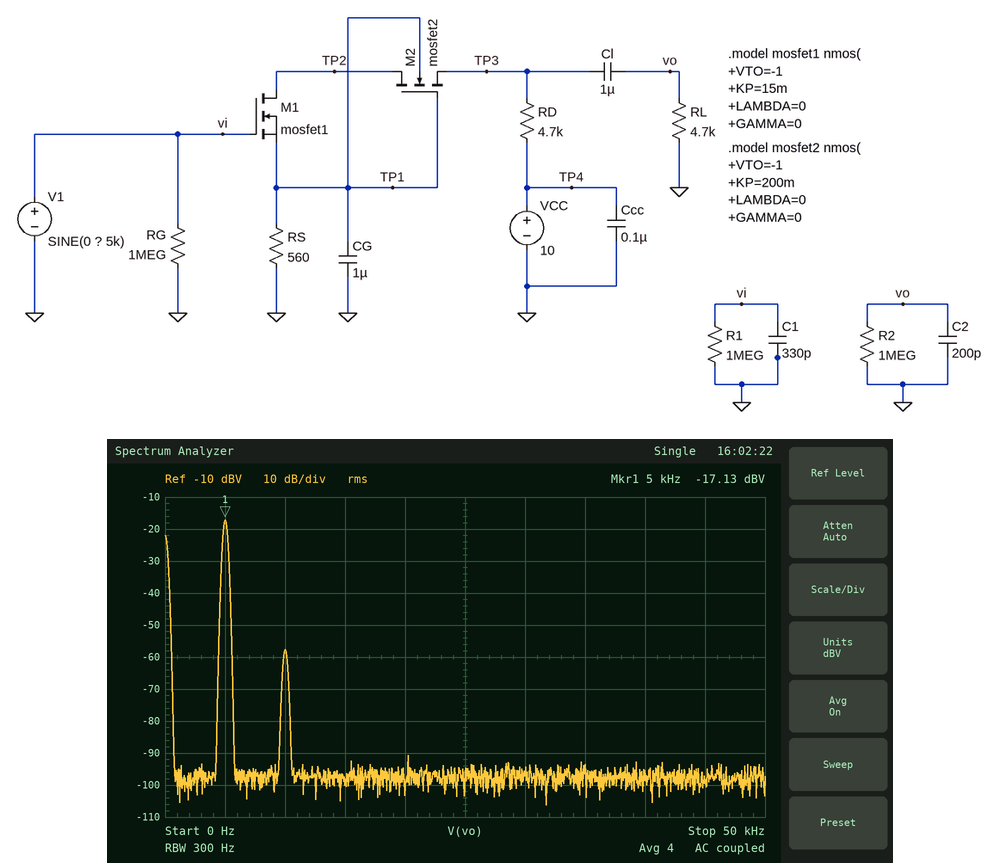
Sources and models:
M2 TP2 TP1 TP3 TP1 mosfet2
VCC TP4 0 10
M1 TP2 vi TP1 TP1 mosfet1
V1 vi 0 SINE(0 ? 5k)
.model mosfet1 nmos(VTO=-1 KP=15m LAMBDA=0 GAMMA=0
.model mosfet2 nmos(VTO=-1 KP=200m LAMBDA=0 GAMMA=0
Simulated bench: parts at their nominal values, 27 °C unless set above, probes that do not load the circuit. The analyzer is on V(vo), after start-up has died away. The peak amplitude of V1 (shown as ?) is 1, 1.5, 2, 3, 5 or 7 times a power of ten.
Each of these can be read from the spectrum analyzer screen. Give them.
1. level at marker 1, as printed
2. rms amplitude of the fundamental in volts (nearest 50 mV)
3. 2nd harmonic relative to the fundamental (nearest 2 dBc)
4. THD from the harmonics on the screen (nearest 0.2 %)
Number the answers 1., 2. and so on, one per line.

1. -17.13 dBV
2. 150 mV
3. -40 dBc
4. 1.0 %
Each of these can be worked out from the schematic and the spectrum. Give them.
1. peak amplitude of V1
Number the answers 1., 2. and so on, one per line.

1. 15 mV
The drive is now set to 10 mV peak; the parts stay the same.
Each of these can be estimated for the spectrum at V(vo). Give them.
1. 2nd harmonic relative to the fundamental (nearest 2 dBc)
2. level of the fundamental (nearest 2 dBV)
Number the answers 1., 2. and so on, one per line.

1. -44 dBc
2. -20 dBV
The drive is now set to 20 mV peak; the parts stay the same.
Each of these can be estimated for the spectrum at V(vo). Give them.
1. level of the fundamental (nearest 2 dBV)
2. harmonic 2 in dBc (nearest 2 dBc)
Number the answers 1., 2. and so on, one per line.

1. -14 dBV
2. -38 dBc
